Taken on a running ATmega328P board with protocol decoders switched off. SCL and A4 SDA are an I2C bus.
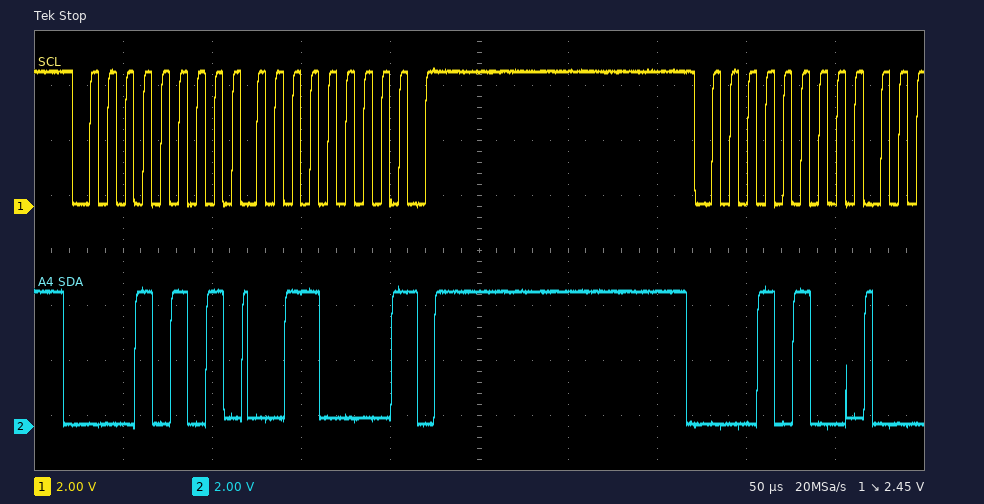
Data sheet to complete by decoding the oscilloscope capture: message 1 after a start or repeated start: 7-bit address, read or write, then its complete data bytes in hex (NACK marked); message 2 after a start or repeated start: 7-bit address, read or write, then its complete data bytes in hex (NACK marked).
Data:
0x0A read: 30 NACK
0x0A write
